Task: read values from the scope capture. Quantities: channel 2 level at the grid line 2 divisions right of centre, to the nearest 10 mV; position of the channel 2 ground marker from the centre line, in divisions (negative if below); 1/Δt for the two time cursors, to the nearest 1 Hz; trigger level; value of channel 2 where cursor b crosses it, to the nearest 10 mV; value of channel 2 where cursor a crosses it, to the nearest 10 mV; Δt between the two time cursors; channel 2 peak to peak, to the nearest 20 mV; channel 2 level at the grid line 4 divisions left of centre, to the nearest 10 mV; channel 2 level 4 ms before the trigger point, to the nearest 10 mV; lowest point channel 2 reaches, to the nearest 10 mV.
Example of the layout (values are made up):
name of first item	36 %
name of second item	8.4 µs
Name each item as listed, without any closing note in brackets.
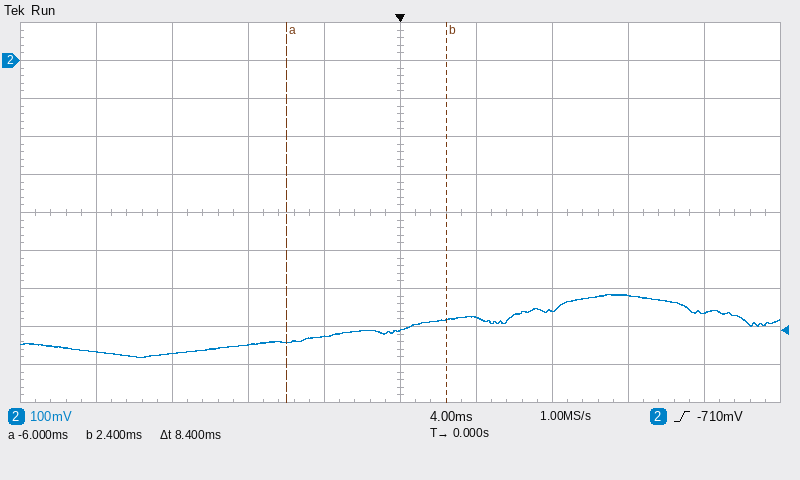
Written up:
channel 2 level at the grid line 2 divisions right of centre, to the nearest 10 mV	-660 mV
position of the channel 2 ground marker from the centre line, in divisions	+4.0 div
1/Δt for the two time cursors, to the nearest 1 Hz	119 Hz
trigger level	-710 mV
value of channel 2 where cursor b crosses it, to the nearest 10 mV	-680 mV
value of channel 2 where cursor a crosses it, to the nearest 10 mV	-740 mV
Δt between the two time cursors	8.4 ms
channel 2 peak to peak, to the nearest 20 mV	160 mV
channel 2 level at the grid line 4 divisions left of centre, to the nearest 10 mV	-770 mV
channel 2 level 4 ms before the trigger point, to the nearest 10 mV	-730 mV
lowest point channel 2 reaches, to the nearest 10 mV	-780 mV
